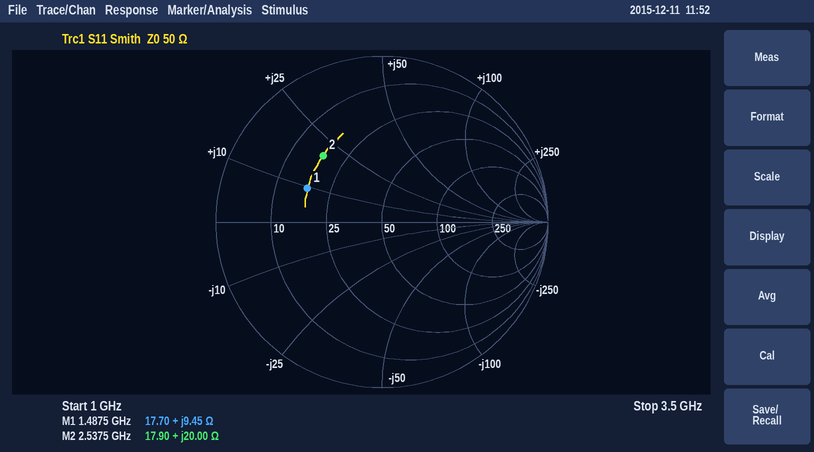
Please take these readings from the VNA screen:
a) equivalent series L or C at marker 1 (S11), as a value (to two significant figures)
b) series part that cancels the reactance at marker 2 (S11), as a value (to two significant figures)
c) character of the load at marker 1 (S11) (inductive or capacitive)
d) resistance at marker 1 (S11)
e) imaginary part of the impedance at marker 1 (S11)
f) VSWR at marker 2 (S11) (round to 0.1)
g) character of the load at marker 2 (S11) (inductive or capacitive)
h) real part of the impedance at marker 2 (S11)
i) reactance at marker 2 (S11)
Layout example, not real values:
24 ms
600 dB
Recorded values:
1.0 nH
3.1 pF
inductive
17.70 Ω
+9.45 Ω
3.3
inductive
17.90 Ω
+20.00 Ω
